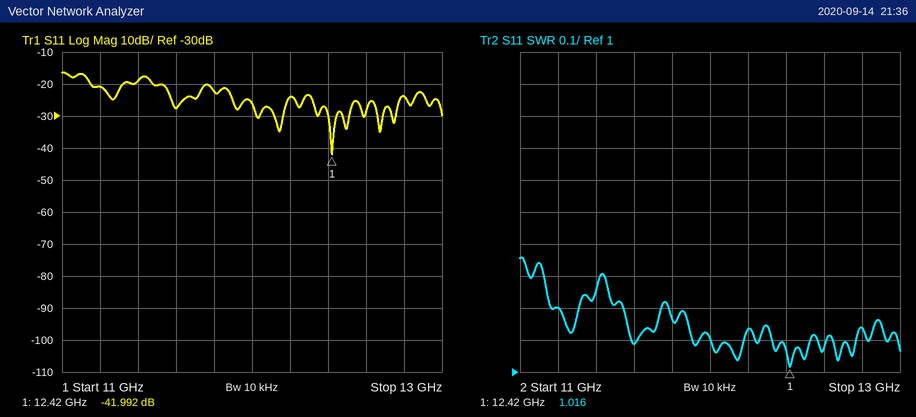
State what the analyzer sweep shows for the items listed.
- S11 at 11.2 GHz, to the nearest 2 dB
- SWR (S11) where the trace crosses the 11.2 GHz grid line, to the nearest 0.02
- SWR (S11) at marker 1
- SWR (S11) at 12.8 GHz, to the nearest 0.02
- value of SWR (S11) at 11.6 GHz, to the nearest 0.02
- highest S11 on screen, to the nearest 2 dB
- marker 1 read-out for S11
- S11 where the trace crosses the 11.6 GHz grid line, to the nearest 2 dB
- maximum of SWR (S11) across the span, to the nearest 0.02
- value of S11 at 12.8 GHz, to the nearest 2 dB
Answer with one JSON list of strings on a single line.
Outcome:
["-20 dB", "1.20", "1.016", "1.14", "1.08", "-16 dB", "-41.992 dB", "-28 dB", "1.36", "-24 dB"]
